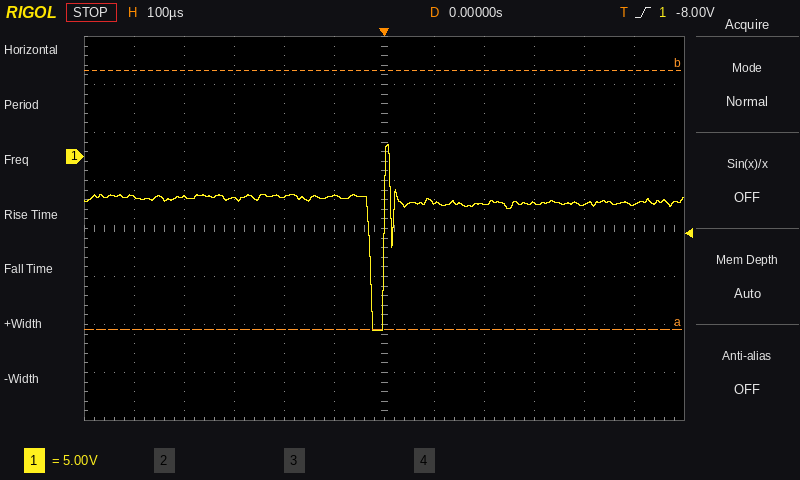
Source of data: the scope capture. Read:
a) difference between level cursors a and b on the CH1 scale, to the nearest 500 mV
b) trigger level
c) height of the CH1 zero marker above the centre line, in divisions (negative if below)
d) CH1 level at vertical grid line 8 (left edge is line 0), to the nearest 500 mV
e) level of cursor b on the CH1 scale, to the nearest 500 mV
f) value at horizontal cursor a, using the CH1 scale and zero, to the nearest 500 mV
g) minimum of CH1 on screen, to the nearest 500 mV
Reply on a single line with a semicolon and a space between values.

27.0 V; -8.00 V; +1.5 div; -5.0 V; 9.0 V; -18.0 V; -18.0 V
